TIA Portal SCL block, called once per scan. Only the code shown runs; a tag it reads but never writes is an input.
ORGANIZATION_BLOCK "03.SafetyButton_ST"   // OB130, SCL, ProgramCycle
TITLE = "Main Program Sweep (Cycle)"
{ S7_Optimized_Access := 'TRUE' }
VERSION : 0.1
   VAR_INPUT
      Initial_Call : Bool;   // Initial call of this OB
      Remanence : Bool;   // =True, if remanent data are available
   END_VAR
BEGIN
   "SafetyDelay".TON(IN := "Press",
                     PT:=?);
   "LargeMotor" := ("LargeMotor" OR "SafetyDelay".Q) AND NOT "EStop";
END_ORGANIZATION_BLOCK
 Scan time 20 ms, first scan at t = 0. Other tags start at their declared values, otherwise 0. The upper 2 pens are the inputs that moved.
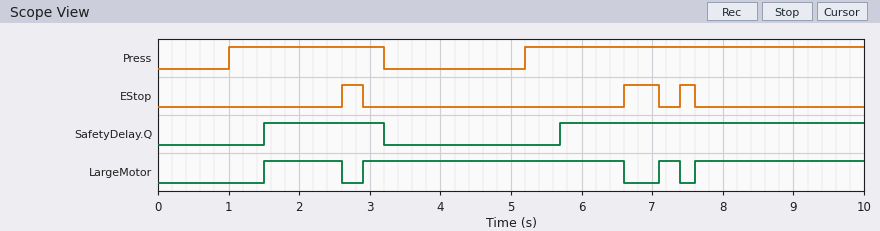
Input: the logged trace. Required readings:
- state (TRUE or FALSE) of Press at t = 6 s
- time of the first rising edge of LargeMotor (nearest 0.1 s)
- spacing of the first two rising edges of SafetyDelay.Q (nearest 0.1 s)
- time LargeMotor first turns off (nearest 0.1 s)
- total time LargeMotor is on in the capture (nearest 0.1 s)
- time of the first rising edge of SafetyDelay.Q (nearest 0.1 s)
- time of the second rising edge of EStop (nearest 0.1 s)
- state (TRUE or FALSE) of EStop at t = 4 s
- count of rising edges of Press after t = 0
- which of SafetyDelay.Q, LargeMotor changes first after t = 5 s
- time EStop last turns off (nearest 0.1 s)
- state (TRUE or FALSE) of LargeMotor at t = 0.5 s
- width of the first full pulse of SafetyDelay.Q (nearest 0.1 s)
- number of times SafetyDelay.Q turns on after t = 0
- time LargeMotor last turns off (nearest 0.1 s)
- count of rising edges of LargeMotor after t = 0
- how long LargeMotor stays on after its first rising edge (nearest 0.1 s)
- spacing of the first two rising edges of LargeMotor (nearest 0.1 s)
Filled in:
TRUE
1.5 s
4.2 s
2.6 s
7.5 s
1.5 s
6.6 s
FALSE
2
SafetyDelay.Q
7.6 s
FALSE
1.7 s
2
7.4 s
4
1.1 s
1.4 s
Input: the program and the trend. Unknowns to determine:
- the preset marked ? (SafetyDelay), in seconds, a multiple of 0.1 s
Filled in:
0.5 s
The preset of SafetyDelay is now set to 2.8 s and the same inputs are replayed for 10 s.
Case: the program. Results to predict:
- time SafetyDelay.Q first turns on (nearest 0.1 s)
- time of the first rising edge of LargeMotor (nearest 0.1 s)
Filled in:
8.0 s
8.0 s
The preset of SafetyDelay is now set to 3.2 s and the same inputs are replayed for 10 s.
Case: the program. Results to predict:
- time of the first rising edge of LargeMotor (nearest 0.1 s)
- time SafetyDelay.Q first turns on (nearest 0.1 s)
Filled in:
8.4 s
8.4 s
